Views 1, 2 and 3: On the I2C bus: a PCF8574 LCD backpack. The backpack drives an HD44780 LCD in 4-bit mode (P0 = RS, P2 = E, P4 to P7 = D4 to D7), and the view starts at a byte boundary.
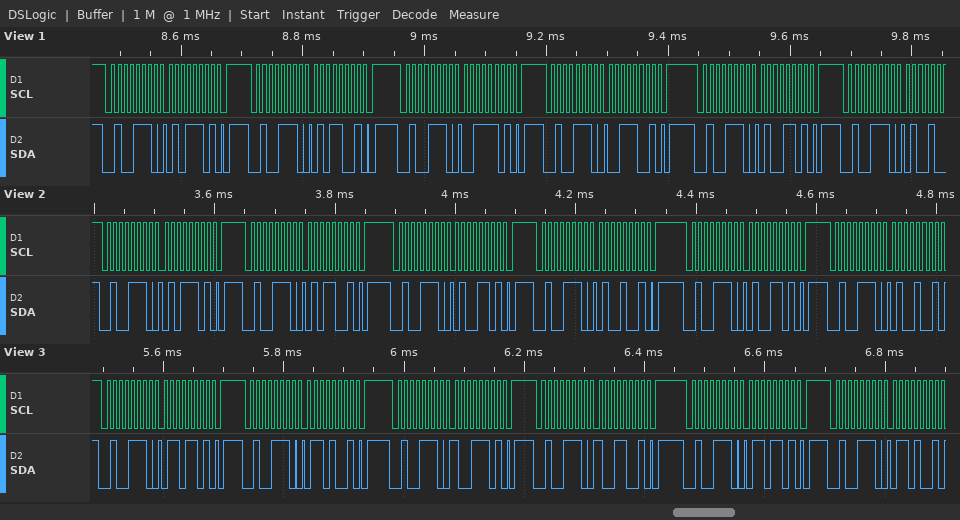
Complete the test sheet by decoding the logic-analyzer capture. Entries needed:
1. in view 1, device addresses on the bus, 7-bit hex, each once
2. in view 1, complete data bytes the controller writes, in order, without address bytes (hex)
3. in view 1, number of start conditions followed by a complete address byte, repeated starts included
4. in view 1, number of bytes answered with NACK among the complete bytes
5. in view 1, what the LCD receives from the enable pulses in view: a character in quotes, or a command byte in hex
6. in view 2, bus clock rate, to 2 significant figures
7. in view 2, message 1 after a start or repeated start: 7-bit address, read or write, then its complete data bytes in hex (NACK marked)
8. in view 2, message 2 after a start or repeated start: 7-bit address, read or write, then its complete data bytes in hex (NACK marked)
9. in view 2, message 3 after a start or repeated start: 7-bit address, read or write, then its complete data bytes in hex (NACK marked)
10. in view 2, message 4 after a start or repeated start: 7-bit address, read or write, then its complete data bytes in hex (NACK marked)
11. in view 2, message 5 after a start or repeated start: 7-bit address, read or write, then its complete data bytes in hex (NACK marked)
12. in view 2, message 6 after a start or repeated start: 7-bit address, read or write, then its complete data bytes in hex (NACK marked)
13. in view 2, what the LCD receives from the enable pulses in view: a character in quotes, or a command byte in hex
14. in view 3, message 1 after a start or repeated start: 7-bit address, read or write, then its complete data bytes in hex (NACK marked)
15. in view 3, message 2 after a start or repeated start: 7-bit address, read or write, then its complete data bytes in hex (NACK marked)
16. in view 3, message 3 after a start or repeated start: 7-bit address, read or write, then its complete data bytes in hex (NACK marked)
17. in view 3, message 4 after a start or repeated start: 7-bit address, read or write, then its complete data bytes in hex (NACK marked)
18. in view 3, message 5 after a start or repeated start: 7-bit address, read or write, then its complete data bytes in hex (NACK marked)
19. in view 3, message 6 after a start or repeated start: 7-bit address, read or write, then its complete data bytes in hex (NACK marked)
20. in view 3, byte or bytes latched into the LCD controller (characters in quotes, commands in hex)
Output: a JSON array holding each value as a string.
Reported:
["0x27", "5D 59 3D 39 4D", "6", "0", "'S'", "100 kHz", "0x27 write: 5D", "0x27 write: 59", "0x27 write: 4D", "0x27 write: 49", "0x27 write: 4D", "0x27 write: 49", "'T'", "0x27 write: 6D", "0x27 write: 69", "0x27 write: 9D", "0x27 write: 99", "0x27 write: 6D", "0x27 write: 69", "'i'"]
